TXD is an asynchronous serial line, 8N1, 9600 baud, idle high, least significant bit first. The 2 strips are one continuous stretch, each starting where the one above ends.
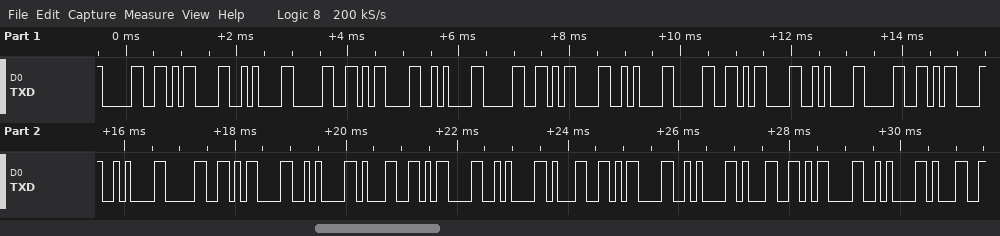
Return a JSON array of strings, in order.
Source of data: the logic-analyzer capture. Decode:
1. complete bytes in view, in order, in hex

["30 0D 0A 30 0D 0A 30 0D 0A 30 0D 0A 30 0D 0A 30 0D 0A 31 0D 0A 31 0D 0A 31 0D 0A 31"]
